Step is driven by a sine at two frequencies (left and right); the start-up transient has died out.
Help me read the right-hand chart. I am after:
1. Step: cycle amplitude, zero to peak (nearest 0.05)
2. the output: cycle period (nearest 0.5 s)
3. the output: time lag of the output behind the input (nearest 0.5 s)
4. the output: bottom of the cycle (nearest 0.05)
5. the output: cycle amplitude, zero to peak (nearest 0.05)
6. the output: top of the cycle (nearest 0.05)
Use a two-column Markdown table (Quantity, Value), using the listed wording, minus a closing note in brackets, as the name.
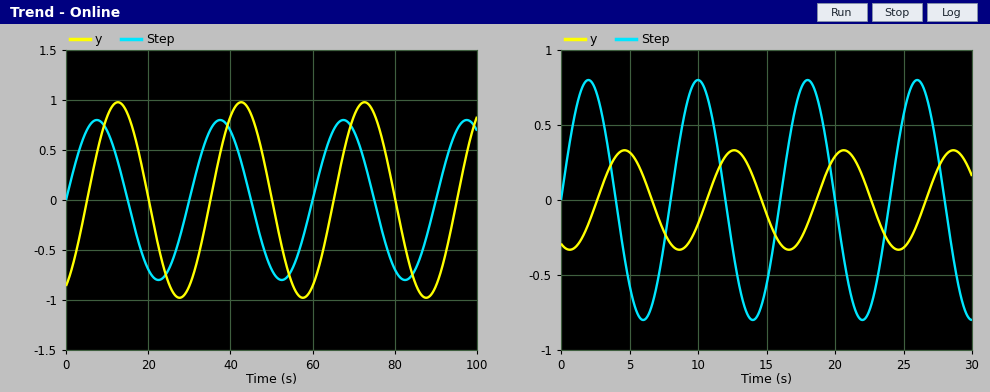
| Quantity | Value |
|---|---|
| Step: cycle amplitude, zero to peak | 0.80 |
| the output: cycle period | 8.0 s |
| the output: time lag of the output behind the input | 2.5 s |
| the output: bottom of the cycle | -0.35 |
| the output: cycle amplitude, zero to peak | 0.35 |
| the output: top of the cycle | 0.35 |
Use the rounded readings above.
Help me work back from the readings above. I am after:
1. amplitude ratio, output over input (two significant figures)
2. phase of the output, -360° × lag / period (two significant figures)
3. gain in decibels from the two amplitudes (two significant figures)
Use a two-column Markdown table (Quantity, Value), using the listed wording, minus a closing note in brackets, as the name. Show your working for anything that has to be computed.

| Quantity | Value |
|---|---|
| amplitude ratio, output over input | 0.35 / 0.8 = 0.44 |
| phase of the output, -360° × lag / period | -360 × 2.5 / 8 = -110° |
| gain in decibels from the two amplitudes | 20 log10(0.35 / 0.8) = -7.2 dB |
